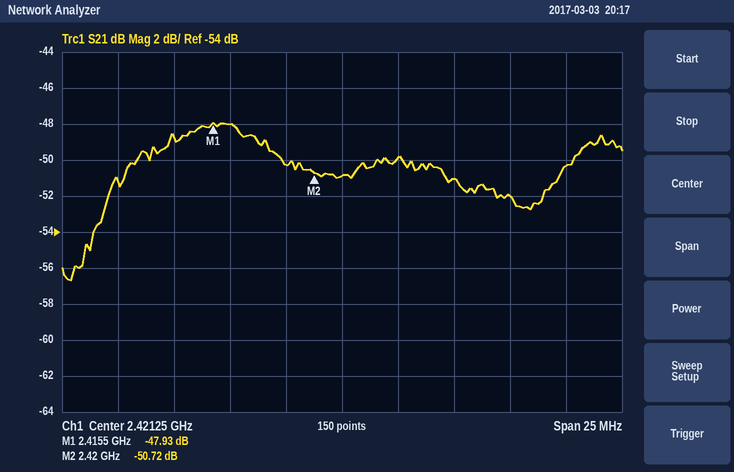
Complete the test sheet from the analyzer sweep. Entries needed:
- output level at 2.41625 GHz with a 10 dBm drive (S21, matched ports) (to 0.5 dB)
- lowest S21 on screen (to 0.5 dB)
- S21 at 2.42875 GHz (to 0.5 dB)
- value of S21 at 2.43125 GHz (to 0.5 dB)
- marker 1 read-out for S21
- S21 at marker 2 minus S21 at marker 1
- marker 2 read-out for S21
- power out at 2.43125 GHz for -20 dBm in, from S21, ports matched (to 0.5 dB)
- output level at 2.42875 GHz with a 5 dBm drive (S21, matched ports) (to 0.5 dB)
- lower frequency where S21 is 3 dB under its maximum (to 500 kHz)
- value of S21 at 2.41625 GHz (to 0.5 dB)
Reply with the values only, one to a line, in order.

-38.0 dBm
-56.5 dB
-52.0 dB
-50.5 dB
-47.93 dB
-2.79 dB
-50.72 dB
-70.5 dBm
-47.0 dBm
2.4115 GHz
-48.0 dB
